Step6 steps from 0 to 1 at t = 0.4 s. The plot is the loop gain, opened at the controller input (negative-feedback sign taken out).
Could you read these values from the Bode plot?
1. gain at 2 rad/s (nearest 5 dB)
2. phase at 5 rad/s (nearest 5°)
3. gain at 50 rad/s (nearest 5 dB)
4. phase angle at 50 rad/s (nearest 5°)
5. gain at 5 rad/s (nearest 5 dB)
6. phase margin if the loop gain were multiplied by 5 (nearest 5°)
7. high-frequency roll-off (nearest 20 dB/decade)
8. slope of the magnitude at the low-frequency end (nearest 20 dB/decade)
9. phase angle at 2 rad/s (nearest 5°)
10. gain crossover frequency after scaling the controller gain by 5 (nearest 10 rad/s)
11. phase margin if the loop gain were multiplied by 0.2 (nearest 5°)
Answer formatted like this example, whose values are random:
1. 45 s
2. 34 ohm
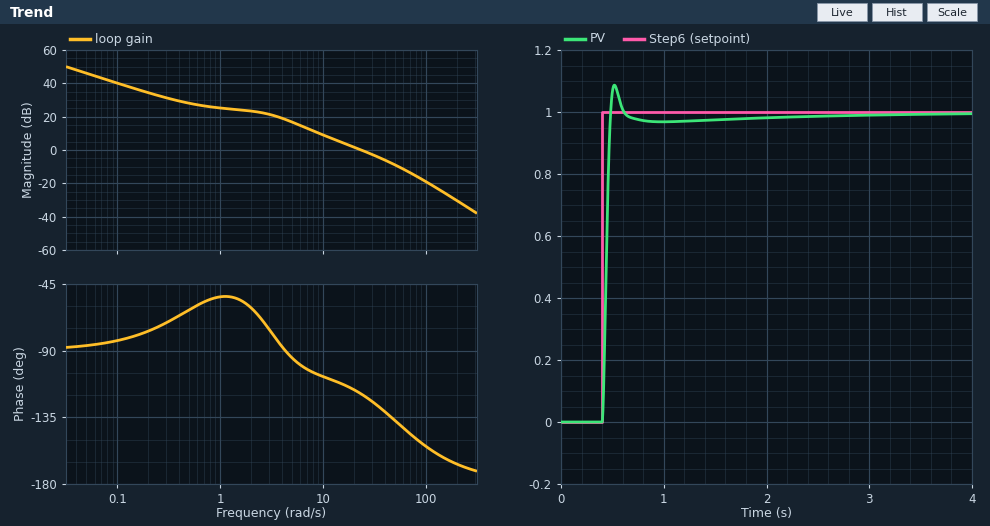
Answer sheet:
1. 25 dB
2. -95°
3. -10 dB
4. -135°
5. 15 dB
6. 35°
7. -40 dB/decade
8. -20 dB/decade
9. -60°
10. 70 rad/s
11. 80°
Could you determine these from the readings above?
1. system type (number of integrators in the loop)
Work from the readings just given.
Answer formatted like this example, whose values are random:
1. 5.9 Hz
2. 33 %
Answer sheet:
1. 1
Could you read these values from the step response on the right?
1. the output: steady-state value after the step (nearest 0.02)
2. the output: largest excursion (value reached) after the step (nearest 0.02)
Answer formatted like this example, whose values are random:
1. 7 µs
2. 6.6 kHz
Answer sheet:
1. 1.00
2. 1.08
